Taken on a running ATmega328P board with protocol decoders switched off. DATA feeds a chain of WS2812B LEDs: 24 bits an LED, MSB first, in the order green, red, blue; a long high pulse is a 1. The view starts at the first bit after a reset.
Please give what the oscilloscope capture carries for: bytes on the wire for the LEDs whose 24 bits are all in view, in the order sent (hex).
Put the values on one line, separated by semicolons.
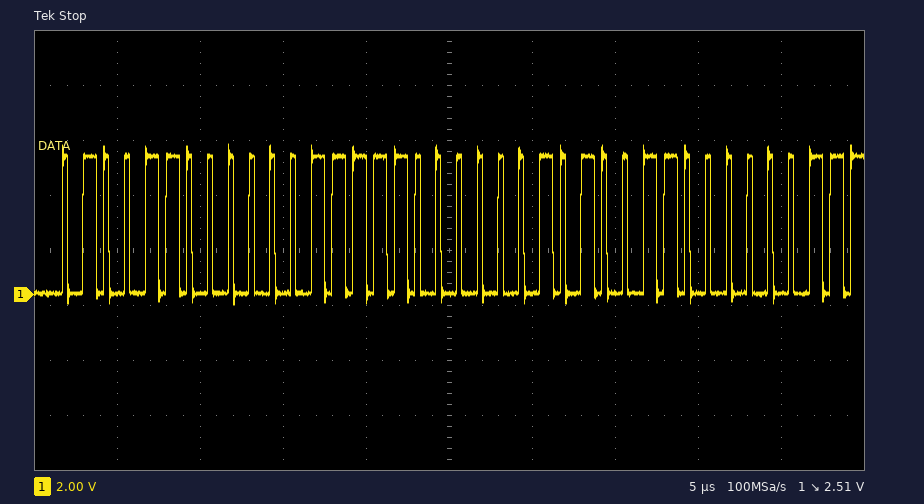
4C 0F 81
